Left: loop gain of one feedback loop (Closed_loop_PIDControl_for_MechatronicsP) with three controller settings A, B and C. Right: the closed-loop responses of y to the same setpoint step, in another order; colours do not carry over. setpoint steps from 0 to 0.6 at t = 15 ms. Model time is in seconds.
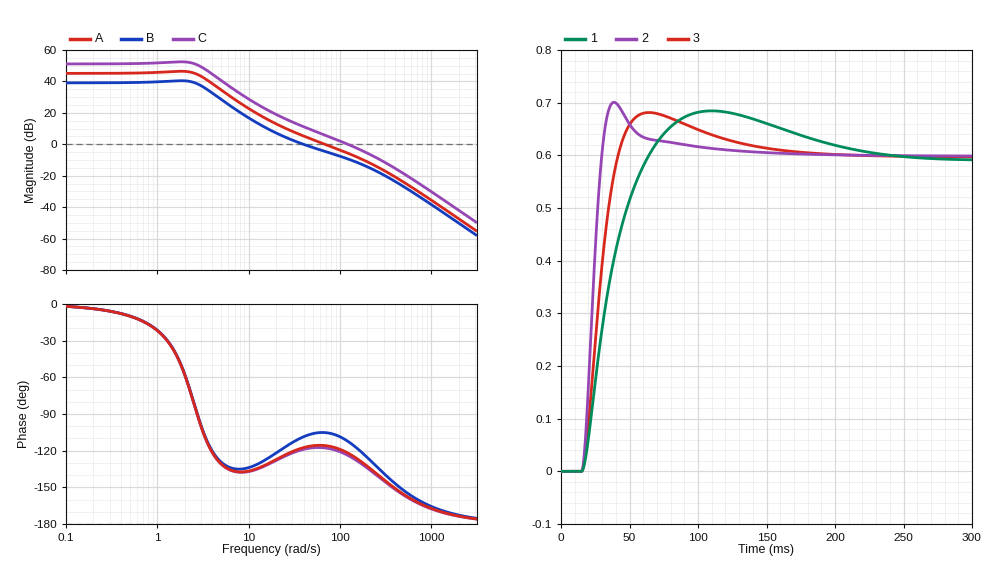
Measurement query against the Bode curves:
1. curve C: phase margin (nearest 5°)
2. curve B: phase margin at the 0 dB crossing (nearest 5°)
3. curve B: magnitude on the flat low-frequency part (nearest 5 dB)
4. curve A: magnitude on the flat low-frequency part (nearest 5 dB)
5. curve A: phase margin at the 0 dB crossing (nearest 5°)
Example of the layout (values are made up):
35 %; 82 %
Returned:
55°; 70°; 40 dB; 45 dB; 65°
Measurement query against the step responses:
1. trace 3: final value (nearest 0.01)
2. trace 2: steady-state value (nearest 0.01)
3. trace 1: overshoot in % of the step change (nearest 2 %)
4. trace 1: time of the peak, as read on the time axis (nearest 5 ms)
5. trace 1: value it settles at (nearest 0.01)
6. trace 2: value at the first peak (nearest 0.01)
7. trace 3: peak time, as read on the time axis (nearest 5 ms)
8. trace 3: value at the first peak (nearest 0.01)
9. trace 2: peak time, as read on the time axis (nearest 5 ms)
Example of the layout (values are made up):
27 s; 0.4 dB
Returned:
0.60; 0.60; 16 %; 110 ms; 0.59; 0.70; 65 ms; 0.68; 40 ms
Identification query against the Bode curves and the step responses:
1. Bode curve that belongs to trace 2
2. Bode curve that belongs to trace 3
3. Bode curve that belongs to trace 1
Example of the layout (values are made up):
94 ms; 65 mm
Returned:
C; A; B
